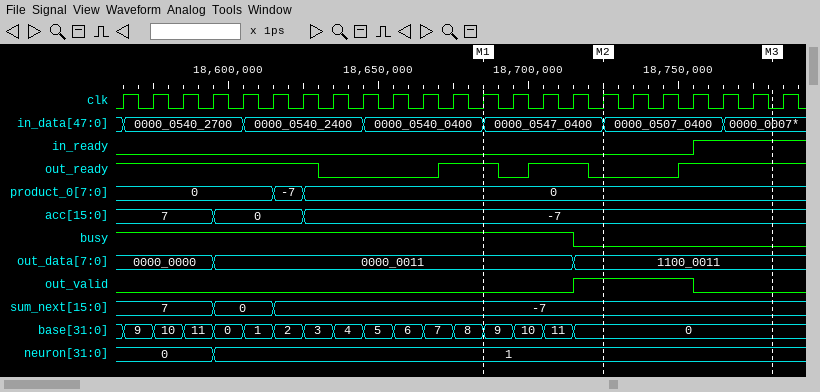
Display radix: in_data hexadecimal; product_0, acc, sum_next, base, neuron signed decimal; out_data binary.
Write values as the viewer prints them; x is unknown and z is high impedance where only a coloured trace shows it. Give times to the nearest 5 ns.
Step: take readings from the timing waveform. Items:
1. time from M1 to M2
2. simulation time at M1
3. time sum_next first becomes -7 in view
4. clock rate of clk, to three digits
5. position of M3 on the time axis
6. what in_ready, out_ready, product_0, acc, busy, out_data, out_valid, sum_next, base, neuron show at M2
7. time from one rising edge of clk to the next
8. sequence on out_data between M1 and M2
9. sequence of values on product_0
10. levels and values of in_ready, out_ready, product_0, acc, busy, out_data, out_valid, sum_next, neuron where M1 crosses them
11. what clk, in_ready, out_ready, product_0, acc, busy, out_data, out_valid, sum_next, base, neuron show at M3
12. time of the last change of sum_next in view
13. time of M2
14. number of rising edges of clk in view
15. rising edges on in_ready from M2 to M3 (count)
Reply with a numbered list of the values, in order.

1. 40 ns
2. 18685 ns
3. 18615 ns
4. 100 MHz
5. 18780 ns
6. in_ready=0, out_ready=0, product_0=0, acc=-7, busy=0, out_data=1100_0011, out_valid=1, sum_next=-7, base=0, neuron=1
7. 10 ns
8. 0000_0011, 1100_0011
9. 0, -7, 0
10. in_ready=0, out_ready=1, product_0=0, acc=-7, busy=1, out_data=0000_0011, out_valid=0, sum_next=-7, neuron=1
11. clk=0, in_ready=1, out_ready=1, product_0=0, acc=-7, busy=0, out_data=1100_0011, out_valid=0, sum_next=-7, base=0, neuron=1
12. 18615 ns
13. 18725 ns
14. 23
15. 1
